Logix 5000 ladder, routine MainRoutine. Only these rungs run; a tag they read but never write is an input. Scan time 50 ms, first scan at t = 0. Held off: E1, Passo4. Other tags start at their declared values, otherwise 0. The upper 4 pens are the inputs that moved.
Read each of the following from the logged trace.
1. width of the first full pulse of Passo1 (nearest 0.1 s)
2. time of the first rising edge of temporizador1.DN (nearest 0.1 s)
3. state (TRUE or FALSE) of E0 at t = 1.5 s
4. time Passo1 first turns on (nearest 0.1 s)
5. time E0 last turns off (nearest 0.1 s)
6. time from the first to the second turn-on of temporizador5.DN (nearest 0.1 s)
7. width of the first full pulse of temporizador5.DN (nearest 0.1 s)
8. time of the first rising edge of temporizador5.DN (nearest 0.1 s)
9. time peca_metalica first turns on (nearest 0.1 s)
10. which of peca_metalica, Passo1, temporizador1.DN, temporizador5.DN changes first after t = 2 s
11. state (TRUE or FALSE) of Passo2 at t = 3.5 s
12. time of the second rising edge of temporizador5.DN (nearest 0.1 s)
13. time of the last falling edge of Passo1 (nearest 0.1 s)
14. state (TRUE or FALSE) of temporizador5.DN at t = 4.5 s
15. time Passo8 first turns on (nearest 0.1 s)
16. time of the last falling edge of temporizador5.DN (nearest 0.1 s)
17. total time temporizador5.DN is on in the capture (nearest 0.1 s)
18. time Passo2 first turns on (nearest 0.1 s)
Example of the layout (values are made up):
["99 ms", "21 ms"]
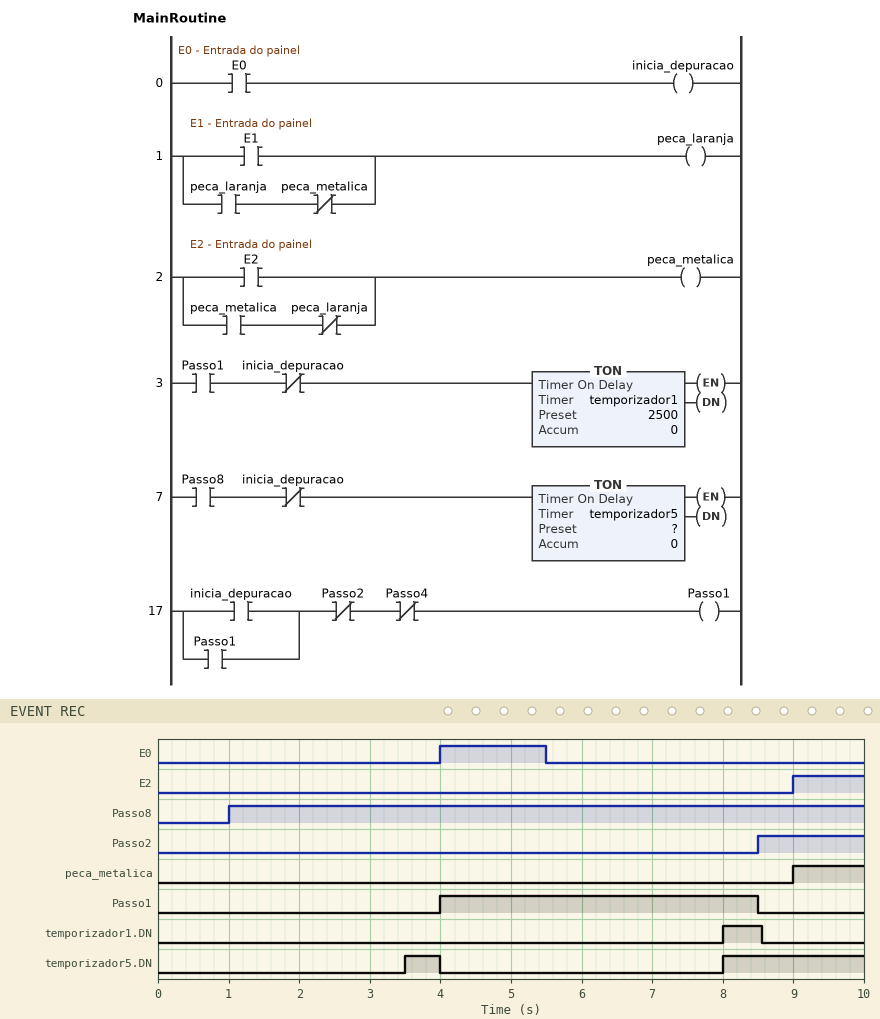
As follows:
["4.5 s", "8.0 s", "FALSE", "4.0 s", "5.5 s", "4.5 s", "0.5 s", "3.5 s", "9.0 s", "temporizador5.DN", "FALSE", "8.0 s", "8.5 s", "FALSE", "1.0 s", "4.0 s", "2.5 s", "8.5 s"]
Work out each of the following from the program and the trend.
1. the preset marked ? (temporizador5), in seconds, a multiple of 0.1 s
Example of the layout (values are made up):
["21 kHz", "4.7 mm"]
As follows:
["2.5 s"]
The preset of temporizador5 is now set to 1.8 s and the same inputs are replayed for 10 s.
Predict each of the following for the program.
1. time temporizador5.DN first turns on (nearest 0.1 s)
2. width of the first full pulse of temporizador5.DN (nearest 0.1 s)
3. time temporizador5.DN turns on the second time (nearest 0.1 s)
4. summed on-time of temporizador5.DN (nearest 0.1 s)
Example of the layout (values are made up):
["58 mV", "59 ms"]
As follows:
["2.8 s", "1.2 s", "7.3 s", "3.9 s"]
